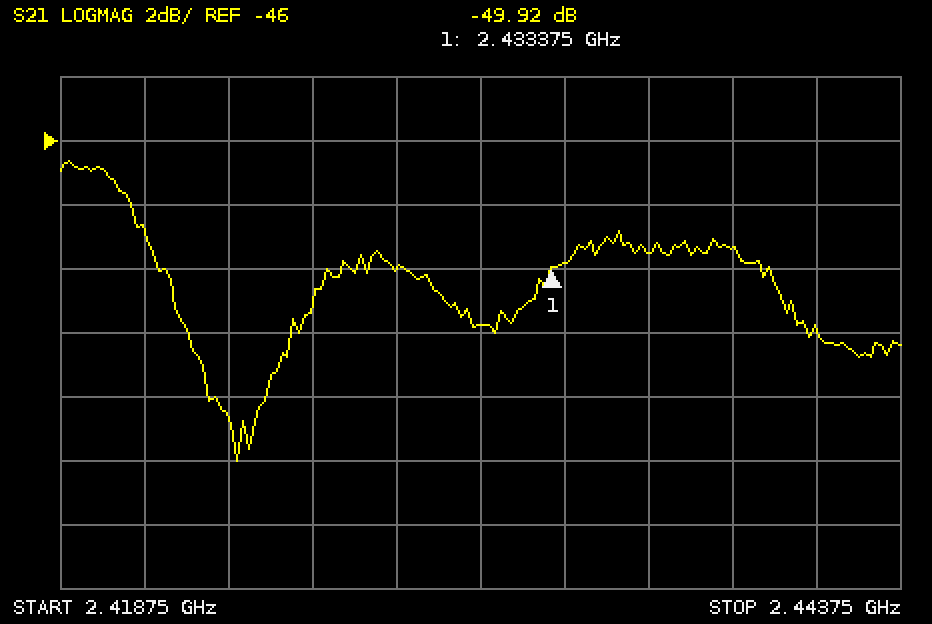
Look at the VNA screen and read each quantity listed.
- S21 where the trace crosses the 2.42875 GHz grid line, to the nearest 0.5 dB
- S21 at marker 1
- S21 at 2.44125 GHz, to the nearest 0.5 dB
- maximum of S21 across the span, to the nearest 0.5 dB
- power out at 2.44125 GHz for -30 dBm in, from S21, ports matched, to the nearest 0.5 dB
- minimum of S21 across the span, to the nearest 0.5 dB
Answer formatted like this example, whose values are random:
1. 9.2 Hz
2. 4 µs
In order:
1. -50.0 dB
2. -49.92 dB
3. -52.0 dB
4. -46.5 dB
5. -82.0 dBm
6. -56.0 dB
